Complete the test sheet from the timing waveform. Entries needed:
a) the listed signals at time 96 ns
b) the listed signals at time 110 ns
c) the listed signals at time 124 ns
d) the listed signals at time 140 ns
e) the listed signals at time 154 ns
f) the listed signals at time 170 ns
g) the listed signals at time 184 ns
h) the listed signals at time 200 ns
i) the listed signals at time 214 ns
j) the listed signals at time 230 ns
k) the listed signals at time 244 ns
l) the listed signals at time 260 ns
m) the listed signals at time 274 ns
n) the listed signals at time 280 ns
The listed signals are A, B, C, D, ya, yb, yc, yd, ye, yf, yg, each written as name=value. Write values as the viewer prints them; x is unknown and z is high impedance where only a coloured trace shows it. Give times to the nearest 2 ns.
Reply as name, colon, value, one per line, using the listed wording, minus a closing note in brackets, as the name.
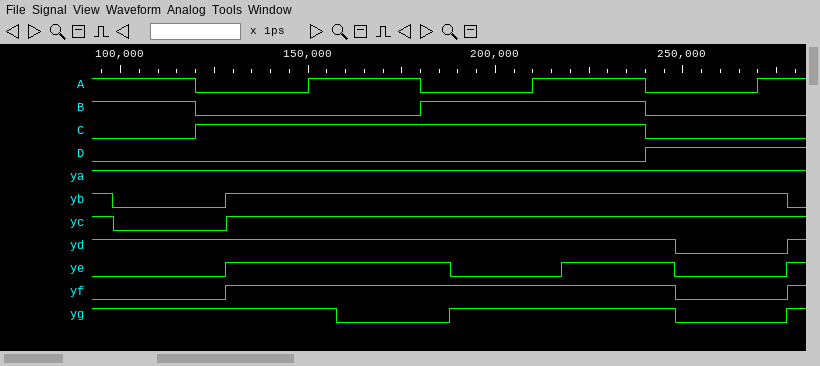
the listed signals at time 96 ns: A=1, B=1, C=0, D=0, ya=1, yb=1, yc=1, yd=1, ye=0, yf=0, yg=1
the listed signals at time 110 ns: A=1, B=1, C=0, D=0, ya=1, yb=0, yc=0, yd=1, ye=0, yf=0, yg=1
the listed signals at time 124 ns: A=0, B=0, C=1, D=0, ya=1, yb=0, yc=0, yd=1, ye=0, yf=0, yg=1
the listed signals at time 140 ns: A=0, B=0, C=1, D=0, ya=1, yb=1, yc=1, yd=1, ye=1, yf=1, yg=1
the listed signals at time 154 ns: A=1, B=0, C=1, D=0, ya=1, yb=1, yc=1, yd=1, ye=1, yf=1, yg=1
the listed signals at time 170 ns: A=1, B=0, C=1, D=0, ya=1, yb=1, yc=1, yd=1, ye=1, yf=1, yg=0
the listed signals at time 184 ns: A=0, B=1, C=1, D=0, ya=1, yb=1, yc=1, yd=1, ye=1, yf=1, yg=0
the listed signals at time 200 ns: A=0, B=1, C=1, D=0, ya=1, yb=1, yc=1, yd=1, ye=0, yf=1, yg=1
the listed signals at time 214 ns: A=1, B=1, C=1, D=0, ya=1, yb=1, yc=1, yd=1, ye=0, yf=1, yg=1
the listed signals at time 230 ns: A=1, B=1, C=1, D=0, ya=1, yb=1, yc=1, yd=1, ye=1, yf=1, yg=1
the listed signals at time 244 ns: A=0, B=0, C=0, D=1, ya=1, yb=1, yc=1, yd=1, ye=1, yf=1, yg=1
the listed signals at time 260 ns: A=0, B=0, C=0, D=1, ya=1, yb=1, yc=1, yd=0, ye=0, yf=0, yg=0
the listed signals at time 274 ns: A=1, B=0, C=0, D=1, ya=1, yb=1, yc=1, yd=0, ye=0, yf=0, yg=0
the listed signals at time 280 ns: A=1, B=0, C=0, D=1, ya=1, yb=0, yc=1, yd=1, ye=1, yf=1, yg=1
